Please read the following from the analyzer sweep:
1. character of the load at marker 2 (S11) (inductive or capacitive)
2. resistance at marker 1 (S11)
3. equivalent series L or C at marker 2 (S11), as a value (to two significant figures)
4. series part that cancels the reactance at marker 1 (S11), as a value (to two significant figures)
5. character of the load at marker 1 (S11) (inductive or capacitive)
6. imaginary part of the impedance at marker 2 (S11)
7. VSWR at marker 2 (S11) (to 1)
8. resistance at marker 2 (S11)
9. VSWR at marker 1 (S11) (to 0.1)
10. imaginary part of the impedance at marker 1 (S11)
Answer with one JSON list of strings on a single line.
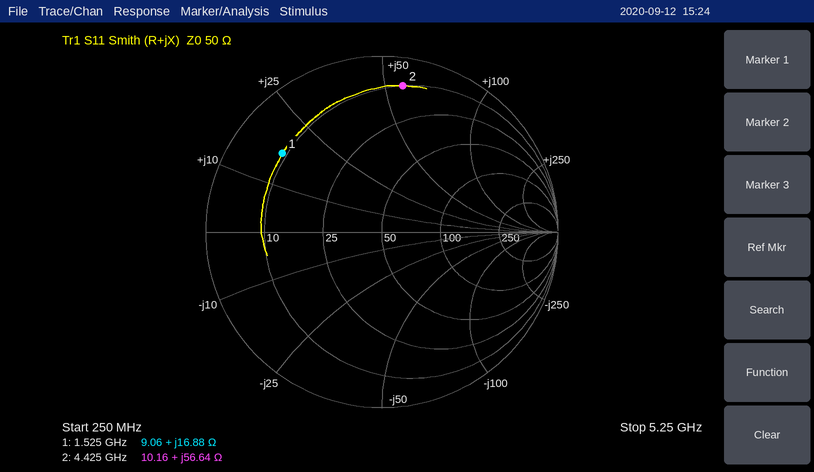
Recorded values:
["inductive", "9.06 Ω", "2.0 nH", "6.2 pF", "inductive", "+56.64 Ω", "11", "10.16 Ω", "6.2", "+16.88 Ω"]
